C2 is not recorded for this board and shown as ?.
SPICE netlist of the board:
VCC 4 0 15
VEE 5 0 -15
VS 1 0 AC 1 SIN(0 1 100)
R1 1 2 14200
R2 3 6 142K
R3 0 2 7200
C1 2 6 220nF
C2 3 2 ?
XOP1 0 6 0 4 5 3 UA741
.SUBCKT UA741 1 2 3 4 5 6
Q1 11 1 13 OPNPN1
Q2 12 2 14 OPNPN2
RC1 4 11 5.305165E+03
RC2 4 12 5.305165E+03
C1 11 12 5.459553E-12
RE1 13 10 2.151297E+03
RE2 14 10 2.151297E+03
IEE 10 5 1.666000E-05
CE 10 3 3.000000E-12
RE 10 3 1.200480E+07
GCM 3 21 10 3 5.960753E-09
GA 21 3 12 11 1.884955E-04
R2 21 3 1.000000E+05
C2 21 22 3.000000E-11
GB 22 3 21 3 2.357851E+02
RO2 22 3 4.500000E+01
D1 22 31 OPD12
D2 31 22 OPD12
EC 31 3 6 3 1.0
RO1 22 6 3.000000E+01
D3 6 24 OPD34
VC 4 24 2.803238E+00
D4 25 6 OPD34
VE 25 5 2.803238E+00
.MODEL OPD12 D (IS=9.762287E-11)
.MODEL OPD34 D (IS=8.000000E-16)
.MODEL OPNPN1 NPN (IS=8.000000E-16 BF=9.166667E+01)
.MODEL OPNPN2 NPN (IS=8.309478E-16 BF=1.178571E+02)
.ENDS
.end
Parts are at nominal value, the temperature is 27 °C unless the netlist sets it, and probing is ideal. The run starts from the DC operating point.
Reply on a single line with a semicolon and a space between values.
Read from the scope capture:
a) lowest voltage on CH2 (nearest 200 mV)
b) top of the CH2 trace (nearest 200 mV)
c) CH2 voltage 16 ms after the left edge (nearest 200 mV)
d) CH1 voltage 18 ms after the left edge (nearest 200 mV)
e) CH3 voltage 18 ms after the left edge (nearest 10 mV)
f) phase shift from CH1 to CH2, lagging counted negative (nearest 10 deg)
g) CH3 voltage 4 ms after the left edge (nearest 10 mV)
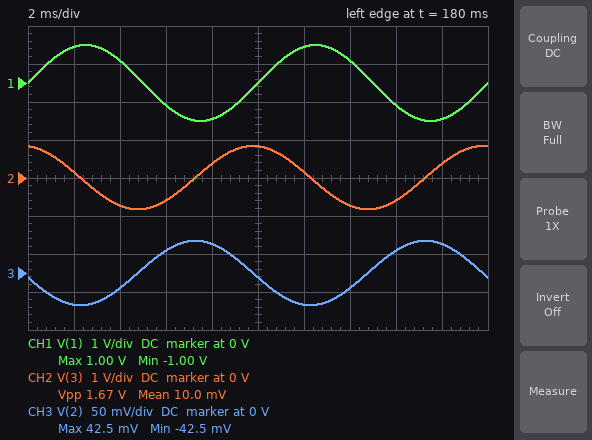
-800 mV; 800 mV; -600 mV; -1.0 V; 40 mV; 100 deg; -20 mV
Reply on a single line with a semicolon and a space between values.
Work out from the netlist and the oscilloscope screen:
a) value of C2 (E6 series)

150 nF
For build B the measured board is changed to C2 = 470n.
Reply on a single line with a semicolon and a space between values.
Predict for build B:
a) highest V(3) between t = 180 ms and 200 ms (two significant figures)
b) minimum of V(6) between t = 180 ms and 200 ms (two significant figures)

260 mV; -1.0 mV
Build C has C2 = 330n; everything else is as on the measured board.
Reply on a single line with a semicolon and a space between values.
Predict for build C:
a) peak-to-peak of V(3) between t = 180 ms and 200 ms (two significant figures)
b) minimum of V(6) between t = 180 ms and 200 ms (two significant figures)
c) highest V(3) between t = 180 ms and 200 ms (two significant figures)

720 mV; -1.0 mV; 370 mV
